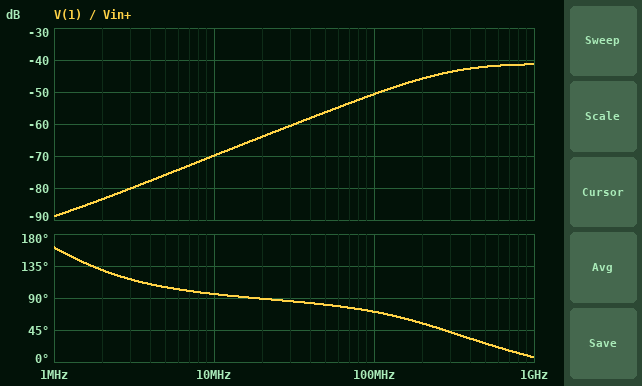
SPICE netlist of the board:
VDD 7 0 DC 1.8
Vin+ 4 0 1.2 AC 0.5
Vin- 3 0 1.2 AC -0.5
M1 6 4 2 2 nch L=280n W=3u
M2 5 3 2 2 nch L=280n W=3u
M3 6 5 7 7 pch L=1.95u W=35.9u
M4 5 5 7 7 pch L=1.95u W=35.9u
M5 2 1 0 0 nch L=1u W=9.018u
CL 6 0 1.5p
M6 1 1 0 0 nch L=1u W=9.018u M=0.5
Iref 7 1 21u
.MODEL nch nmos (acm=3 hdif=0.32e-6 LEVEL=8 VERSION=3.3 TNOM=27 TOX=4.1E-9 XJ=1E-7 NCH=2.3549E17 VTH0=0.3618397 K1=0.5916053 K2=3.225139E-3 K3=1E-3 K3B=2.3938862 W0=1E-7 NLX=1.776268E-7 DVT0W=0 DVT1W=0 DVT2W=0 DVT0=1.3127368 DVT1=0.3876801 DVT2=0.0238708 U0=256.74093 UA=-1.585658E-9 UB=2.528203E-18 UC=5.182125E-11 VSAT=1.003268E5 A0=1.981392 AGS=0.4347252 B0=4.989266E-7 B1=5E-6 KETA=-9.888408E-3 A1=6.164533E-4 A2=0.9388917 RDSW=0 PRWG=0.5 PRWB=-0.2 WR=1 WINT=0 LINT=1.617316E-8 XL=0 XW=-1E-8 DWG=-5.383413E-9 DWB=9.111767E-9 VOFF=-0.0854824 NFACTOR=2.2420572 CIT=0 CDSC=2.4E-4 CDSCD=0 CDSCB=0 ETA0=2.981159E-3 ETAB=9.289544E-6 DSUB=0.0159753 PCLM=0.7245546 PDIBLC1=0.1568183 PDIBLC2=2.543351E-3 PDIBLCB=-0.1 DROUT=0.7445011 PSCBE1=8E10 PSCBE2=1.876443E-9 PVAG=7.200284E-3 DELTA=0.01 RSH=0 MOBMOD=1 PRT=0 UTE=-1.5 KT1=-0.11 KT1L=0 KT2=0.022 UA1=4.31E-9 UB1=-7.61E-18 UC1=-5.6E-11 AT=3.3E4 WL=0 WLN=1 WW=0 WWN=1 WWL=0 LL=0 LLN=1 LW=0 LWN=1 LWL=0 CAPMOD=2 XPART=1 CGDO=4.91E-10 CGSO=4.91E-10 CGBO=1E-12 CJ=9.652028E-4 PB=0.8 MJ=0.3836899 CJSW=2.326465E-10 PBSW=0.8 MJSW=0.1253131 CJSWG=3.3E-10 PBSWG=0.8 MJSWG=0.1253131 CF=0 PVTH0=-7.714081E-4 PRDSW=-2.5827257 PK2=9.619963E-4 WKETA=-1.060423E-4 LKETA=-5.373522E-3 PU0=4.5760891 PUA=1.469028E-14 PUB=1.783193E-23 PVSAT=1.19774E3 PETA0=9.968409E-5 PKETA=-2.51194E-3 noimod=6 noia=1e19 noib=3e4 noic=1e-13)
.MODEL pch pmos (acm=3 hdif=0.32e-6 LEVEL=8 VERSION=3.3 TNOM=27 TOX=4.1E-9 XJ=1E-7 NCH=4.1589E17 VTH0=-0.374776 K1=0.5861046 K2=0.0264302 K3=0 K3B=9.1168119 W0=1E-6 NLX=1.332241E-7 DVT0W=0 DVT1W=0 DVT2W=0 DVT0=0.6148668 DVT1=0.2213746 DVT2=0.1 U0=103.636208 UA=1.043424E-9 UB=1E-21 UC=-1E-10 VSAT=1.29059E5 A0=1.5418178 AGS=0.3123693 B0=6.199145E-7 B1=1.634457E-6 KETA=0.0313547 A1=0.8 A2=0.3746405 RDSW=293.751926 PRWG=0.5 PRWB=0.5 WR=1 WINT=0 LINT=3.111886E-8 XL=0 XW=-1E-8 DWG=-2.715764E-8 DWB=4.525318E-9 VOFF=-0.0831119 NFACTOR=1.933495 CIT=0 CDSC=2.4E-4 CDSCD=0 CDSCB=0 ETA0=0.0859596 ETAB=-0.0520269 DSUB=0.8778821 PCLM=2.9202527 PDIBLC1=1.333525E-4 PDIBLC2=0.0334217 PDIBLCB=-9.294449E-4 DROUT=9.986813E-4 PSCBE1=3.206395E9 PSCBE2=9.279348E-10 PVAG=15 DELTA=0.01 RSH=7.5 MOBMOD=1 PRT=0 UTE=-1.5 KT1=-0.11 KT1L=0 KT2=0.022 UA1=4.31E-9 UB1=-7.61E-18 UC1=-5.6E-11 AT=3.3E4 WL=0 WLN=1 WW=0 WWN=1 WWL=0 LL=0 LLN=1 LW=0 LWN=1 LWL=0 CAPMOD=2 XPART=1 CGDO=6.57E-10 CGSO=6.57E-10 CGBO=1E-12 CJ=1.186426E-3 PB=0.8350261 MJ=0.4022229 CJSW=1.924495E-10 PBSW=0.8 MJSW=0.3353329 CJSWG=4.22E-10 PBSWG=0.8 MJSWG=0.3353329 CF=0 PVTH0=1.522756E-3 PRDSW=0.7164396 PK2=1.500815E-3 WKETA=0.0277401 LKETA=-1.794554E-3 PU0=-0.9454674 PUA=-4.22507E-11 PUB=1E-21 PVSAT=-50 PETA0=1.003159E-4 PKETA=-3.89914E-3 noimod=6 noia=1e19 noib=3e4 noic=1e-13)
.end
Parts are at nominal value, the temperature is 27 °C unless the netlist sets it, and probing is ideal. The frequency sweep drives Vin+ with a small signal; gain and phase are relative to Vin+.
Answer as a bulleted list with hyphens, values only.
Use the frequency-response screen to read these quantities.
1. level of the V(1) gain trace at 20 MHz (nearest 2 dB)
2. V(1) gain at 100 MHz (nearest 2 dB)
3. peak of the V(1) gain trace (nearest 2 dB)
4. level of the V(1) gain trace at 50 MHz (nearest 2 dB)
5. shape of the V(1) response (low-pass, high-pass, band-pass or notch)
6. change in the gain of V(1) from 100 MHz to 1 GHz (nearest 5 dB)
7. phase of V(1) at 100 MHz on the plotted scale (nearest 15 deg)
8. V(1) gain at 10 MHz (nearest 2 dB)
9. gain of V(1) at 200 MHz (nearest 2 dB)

- -64 dB
- -50 dB
- -42 dB
- -56 dB
- high-pass
- 10 dB
- 75 deg
- -70 dB
- -46 dB
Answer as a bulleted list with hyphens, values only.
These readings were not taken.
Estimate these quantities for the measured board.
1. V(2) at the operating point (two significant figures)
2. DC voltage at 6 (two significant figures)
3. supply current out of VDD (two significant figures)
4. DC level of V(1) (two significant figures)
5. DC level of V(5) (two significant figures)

- 610 mV
- 1.2 V
- 63 µA
- 610 mV
- 1.2 V
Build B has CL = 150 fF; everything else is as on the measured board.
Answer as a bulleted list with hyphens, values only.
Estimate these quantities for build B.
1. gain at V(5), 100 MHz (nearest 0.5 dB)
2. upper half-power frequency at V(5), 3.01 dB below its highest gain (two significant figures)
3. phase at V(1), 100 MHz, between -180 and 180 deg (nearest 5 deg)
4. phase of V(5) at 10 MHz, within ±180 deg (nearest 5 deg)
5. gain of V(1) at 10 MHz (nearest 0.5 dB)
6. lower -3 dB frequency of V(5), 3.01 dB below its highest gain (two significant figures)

- -10.5 dB
- 42 MHz
- 75 deg
- 0 deg
- -69.0 dB
- 3.2 MHz
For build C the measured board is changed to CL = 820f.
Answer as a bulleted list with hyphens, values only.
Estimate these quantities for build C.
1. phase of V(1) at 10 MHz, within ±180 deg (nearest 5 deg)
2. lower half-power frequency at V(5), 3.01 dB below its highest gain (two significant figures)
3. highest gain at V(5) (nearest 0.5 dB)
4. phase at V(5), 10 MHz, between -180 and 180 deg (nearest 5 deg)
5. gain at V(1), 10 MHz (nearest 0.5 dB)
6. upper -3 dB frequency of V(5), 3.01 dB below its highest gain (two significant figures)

- 100 deg
- 960 kHz
- 0 dB
- -10 deg
- -70.0 dB
- 35 MHz
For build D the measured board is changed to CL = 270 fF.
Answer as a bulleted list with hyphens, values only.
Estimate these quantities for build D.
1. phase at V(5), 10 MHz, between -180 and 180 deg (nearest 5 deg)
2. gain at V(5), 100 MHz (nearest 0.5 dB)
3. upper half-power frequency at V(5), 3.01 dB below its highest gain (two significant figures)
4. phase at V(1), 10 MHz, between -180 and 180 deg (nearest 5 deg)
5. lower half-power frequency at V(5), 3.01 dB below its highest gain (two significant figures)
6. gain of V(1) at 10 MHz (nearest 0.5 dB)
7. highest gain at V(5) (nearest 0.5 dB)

- -5 deg
- -10.0 dB
- 39 MHz
- 120 deg
- 2.3 MHz
- -69.5 dB
- -1.0 dB
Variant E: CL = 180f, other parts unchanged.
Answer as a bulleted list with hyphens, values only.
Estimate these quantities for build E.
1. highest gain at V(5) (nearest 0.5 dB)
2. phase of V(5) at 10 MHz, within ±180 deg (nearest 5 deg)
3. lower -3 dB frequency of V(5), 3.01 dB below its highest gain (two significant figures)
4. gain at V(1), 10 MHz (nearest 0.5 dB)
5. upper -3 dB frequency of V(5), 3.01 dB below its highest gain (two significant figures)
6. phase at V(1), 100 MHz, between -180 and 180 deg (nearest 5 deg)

- -1.5 dB
- 0 deg
- 2.9 MHz
- -69.0 dB
- 41 MHz
- 75 deg
